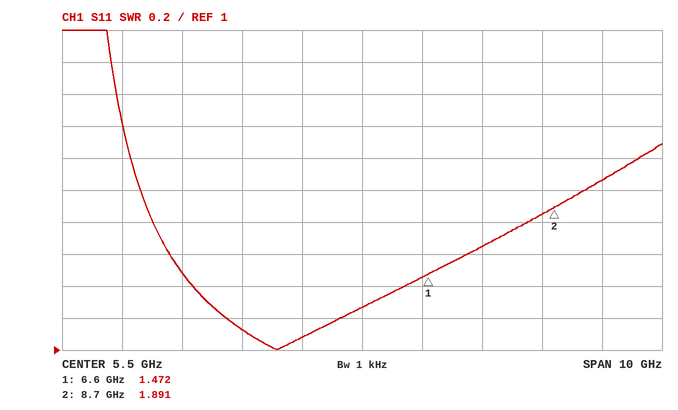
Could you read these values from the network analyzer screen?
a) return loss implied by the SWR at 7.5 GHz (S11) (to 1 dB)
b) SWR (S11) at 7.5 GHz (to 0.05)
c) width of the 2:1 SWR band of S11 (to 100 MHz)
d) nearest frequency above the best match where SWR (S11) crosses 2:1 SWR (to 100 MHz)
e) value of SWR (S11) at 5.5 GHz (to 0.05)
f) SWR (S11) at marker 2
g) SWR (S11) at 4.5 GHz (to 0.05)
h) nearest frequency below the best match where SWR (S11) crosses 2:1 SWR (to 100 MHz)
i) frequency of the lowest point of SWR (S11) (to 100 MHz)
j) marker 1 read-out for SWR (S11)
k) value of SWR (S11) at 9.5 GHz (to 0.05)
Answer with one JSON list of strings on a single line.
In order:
["12 dB", "1.65", "7.4 GHz", "9.2 GHz", "1.25", "1.891", "1.10", "1.8 GHz", "4.1 GHz", "1.472", "2.05"]
